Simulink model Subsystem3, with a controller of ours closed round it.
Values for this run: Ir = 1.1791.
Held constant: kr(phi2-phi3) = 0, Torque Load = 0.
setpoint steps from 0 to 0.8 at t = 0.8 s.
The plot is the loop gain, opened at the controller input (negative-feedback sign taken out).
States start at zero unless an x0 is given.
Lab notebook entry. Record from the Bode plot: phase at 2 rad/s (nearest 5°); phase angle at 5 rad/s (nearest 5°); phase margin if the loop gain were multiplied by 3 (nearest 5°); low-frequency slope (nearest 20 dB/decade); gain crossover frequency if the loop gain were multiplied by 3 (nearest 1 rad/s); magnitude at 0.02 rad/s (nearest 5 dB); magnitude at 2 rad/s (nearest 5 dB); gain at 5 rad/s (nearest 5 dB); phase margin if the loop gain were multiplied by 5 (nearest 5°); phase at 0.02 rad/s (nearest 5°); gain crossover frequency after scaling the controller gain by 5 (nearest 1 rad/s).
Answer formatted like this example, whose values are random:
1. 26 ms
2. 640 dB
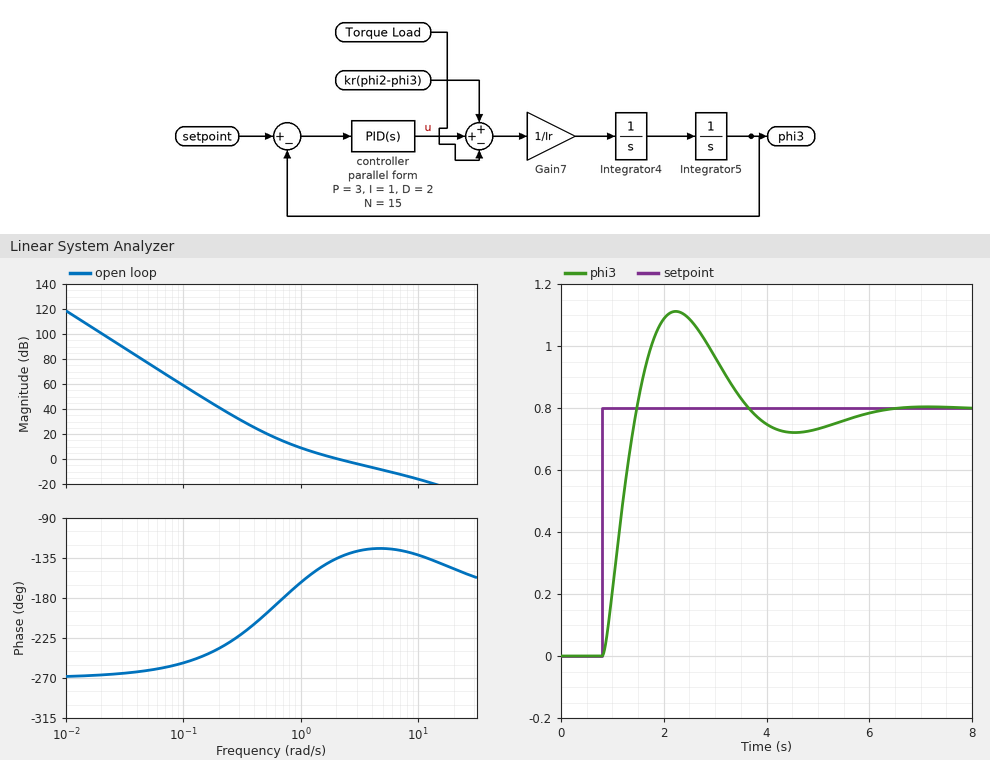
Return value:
1. -135°
2. -125°
3. 55°
4. -60 dB/decade
5. 5 rad/s
6. 100 dB
7. 0 dB
8. -10 dB
9. 50°
10. -265°
11. 8 rad/s
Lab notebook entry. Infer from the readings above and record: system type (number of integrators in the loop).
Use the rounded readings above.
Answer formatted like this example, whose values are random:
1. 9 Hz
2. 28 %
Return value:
1. 3
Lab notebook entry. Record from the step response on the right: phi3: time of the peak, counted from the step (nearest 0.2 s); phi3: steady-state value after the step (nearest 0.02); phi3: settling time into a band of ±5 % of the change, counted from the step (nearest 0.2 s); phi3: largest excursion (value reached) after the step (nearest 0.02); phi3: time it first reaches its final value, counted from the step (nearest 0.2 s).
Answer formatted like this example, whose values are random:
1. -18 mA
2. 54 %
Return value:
1. 1.4 s
2. 0.80
3. 4.8 s
4. 1.12
5. 0.6 s
